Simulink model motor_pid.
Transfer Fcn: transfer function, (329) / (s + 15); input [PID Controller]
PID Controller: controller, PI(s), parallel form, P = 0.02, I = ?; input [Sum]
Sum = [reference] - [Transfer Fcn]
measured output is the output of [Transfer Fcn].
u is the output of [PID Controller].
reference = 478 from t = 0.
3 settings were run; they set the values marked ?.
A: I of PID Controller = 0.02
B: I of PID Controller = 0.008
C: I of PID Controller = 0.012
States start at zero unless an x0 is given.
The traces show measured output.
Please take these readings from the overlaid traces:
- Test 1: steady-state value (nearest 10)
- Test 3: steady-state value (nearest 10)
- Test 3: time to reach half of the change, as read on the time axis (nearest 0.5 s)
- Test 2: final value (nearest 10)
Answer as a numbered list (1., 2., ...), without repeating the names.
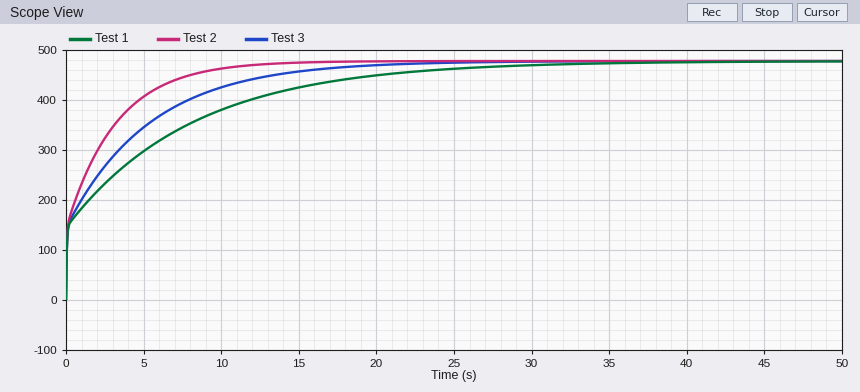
1. 480
2. 480
3. 2.0 s
4. 480
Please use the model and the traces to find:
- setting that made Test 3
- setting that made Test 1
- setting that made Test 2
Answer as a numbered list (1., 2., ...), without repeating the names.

1. C
2. B
3. A
